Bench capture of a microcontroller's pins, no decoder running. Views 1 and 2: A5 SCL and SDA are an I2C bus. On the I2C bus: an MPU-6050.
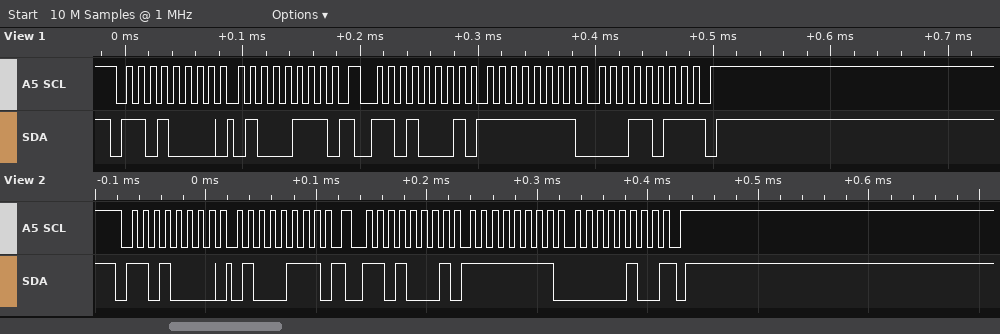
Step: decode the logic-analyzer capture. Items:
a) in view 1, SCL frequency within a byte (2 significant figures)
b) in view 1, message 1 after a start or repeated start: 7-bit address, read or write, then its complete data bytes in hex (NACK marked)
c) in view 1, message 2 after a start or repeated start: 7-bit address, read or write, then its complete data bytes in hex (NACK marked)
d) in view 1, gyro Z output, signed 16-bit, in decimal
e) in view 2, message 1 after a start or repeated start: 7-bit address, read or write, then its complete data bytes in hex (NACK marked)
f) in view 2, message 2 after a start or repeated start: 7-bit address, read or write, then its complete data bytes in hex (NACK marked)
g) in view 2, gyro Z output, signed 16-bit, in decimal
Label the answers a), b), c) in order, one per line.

a) 100 kHz
b) 0x68 write: 47
c) 0x68 read: FF 1B NACK
d) -229
e) 0x68 write: 47
f) 0x68 read: FF 04 NACK
g) -252
